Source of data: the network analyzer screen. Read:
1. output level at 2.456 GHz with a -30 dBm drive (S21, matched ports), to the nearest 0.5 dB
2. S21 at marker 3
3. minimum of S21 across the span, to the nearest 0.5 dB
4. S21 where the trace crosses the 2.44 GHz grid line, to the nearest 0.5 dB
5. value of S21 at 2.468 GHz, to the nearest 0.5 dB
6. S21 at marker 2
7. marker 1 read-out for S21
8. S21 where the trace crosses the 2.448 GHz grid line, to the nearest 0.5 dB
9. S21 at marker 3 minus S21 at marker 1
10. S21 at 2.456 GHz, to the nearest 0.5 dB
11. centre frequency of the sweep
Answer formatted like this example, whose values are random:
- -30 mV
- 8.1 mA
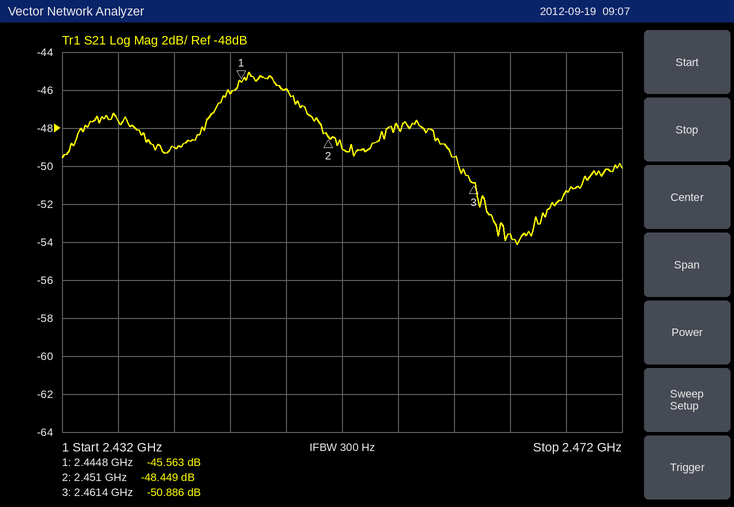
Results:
- -78.0 dBm
- -50.886 dB
- -54.0 dB
- -49.0 dB
- -51.5 dB
- -48.449 dB
- -45.563 dB
- -46.0 dB
- -5.323 dB
- -48.0 dB
- 2.452 GHz
